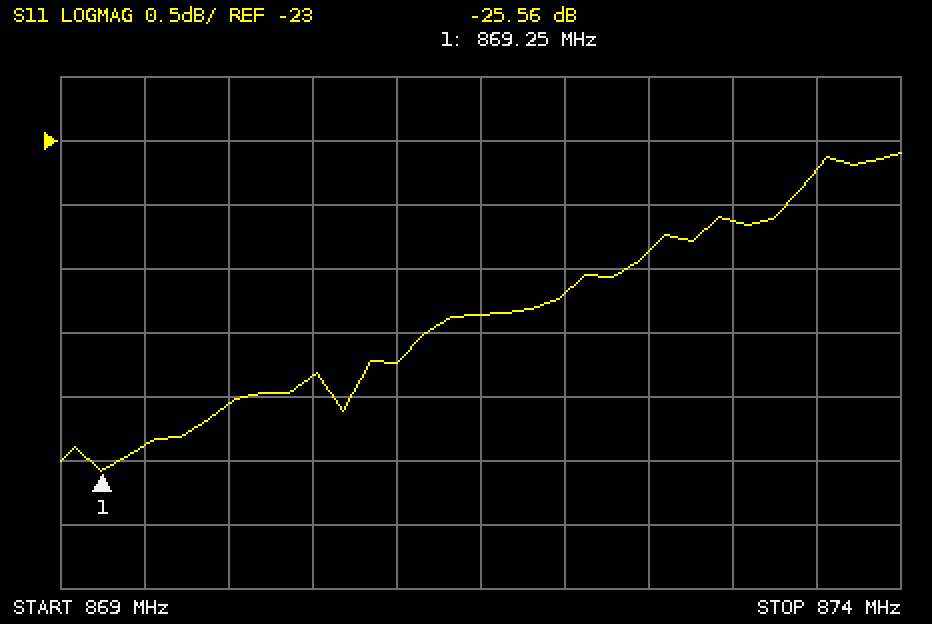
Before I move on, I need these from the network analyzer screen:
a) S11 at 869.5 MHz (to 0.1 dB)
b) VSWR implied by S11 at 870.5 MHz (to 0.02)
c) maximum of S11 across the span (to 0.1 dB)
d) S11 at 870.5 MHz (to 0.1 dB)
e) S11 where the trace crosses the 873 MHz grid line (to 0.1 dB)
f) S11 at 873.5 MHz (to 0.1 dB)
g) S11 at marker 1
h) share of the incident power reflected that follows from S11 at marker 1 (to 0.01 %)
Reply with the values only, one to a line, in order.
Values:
-25.4 dB
1.12
-23.1 dB
-24.8 dB
-23.6 dB
-23.2 dB
-25.56 dB
0.28 %
